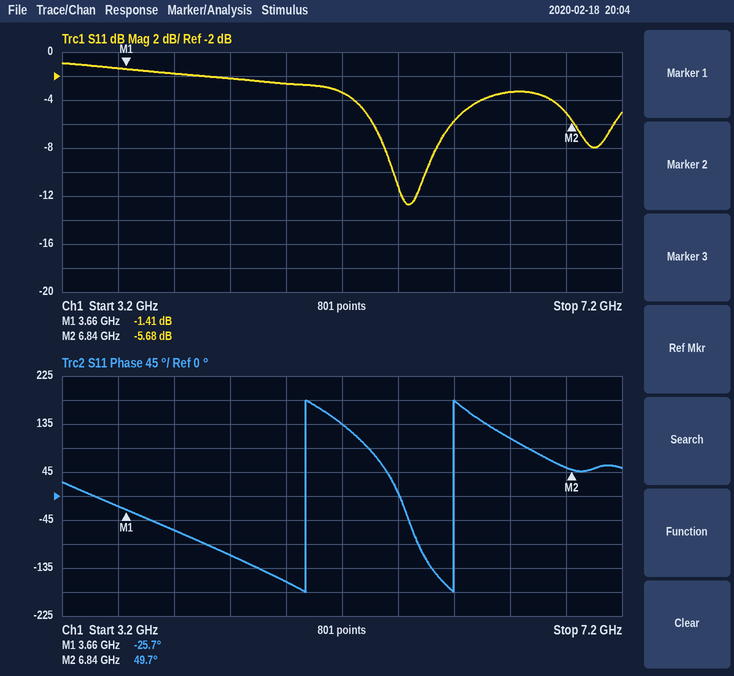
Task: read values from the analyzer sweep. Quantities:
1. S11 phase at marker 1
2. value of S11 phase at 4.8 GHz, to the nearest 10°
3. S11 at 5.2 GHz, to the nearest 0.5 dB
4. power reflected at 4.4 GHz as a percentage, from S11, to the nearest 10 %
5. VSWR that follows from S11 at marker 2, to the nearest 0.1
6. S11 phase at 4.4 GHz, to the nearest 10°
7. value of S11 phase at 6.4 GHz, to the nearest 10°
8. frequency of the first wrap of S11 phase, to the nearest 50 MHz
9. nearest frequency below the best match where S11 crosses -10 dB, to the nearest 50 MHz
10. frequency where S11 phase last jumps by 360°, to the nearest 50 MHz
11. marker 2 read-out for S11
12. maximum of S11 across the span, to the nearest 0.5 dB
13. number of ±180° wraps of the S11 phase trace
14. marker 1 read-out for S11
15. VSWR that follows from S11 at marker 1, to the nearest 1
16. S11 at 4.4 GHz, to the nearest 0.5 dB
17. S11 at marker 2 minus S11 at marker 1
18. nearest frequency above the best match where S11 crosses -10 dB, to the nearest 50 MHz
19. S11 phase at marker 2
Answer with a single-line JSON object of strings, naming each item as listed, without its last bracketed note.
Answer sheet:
{"S11 phase at marker 1": "-25.7°", "value of S11 phase at 4.8 GHz, to the nearest 10°": "-160°", "S11 at 5.2 GHz, to the nearest 0.5 dB": "-3.5 dB", "power reflected at 4.4 GHz as a percentage, from S11, to the nearest 10 %": "60 %", "VSWR that follows from S11 at marker 2, to the nearest 0.1": "3.2", "S11 phase at 4.4 GHz, to the nearest 10°": "-110°", "value of S11 phase at 6.4 GHz, to the nearest 10°": "110°", "frequency of the first wrap of S11 phase, to the nearest 50 MHz": "4.95 GHz", "nearest frequency below the best match where S11 crosses -10 dB, to the nearest 50 MHz": "5.55 GHz", "frequency where S11 phase last jumps by 360°, to the nearest 50 MHz": "6.00 GHz", "marker 2 read-out for S11": "-5.68 dB", "maximum of S11 across the span, to the nearest 0.5 dB": "-1.0 dB", "number of ±180° wraps of the S11 phase trace": "2", "marker 1 read-out for S11": "-1.41 dB", "VSWR that follows from S11 at marker 1, to the nearest 1": "12", "S11 at 4.4 GHz, to the nearest 0.5 dB": "-2.0 dB", "S11 at marker 2 minus S11 at marker 1": "-4.27 dB", "nearest frequency above the best match where S11 crosses -10 dB, to the nearest 50 MHz": "5.80 GHz", "S11 phase at marker 2": "49.7°"}
